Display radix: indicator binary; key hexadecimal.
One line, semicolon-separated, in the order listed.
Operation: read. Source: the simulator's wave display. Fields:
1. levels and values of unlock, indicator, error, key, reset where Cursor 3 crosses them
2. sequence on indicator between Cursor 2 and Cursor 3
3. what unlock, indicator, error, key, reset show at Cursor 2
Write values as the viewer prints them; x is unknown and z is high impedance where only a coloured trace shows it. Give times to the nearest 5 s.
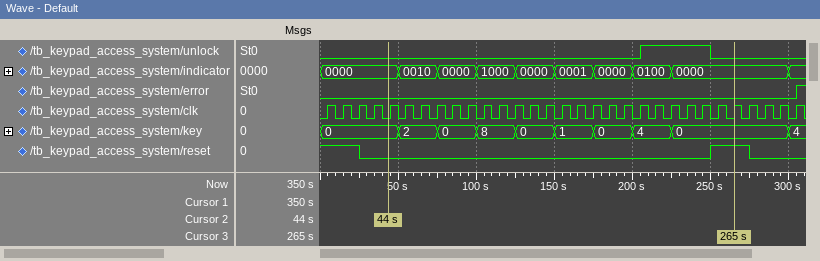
unlock=0, indicator=0000, error=0, key=0, reset=1; 0000, 0010, 0000, 1000, 0000, 0001, 0000, 0100, 0000; unlock=0, indicator=0000, error=0, key=0, reset=0
